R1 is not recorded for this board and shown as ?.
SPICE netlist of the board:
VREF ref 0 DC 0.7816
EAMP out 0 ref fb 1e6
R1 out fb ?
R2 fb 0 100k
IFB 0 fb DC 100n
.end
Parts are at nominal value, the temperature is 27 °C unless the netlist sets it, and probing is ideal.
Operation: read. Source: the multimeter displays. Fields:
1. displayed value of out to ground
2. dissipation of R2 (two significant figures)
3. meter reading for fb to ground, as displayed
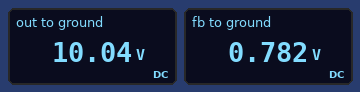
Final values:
10.04 V
6.1 µW
0.782 V
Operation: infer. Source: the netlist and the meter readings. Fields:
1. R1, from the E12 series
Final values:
1.2 MΩ
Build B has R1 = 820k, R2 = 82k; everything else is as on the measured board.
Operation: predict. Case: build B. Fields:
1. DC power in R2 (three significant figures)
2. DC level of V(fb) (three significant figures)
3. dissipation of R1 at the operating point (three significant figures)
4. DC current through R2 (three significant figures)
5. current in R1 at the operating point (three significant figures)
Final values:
7.45 µW
782 mV
72.9 µW
9.53 µA
9.43 µA
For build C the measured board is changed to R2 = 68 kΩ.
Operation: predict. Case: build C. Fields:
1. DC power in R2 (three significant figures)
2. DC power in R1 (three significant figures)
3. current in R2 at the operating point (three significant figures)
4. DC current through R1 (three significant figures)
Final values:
8.98 µW
156 µW
11.5 µA
11.4 µA
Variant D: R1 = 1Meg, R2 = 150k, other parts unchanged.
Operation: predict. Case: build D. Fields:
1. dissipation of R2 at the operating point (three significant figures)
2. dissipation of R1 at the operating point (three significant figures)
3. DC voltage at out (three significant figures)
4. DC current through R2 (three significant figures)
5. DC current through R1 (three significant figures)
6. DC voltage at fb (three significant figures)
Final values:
4.07 µW
26.1 µW
5.89 V
5.21 µA
5.11 µA
782 mV
